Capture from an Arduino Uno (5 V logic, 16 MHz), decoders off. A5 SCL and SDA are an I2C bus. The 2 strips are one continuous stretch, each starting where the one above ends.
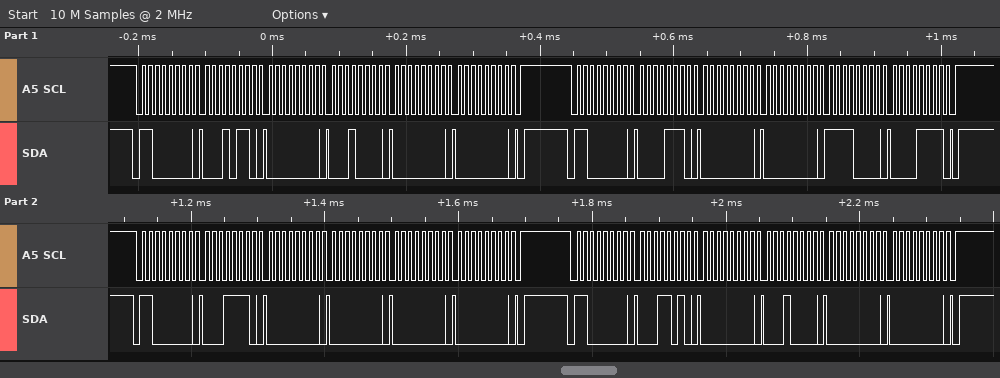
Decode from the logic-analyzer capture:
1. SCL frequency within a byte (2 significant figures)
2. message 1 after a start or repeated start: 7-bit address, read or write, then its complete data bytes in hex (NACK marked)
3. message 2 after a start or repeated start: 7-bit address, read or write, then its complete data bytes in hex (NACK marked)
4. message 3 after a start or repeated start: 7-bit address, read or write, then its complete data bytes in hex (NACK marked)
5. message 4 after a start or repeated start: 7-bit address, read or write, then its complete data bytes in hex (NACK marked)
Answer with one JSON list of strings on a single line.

["100 kHz", "0x60 write: 16 00 10 00 00", "0x60 write: 0E 00 00 F0 0F", "0x60 write: 1E 00 00 00 00", "0x60 write: 1A 00 10 00 00"]
